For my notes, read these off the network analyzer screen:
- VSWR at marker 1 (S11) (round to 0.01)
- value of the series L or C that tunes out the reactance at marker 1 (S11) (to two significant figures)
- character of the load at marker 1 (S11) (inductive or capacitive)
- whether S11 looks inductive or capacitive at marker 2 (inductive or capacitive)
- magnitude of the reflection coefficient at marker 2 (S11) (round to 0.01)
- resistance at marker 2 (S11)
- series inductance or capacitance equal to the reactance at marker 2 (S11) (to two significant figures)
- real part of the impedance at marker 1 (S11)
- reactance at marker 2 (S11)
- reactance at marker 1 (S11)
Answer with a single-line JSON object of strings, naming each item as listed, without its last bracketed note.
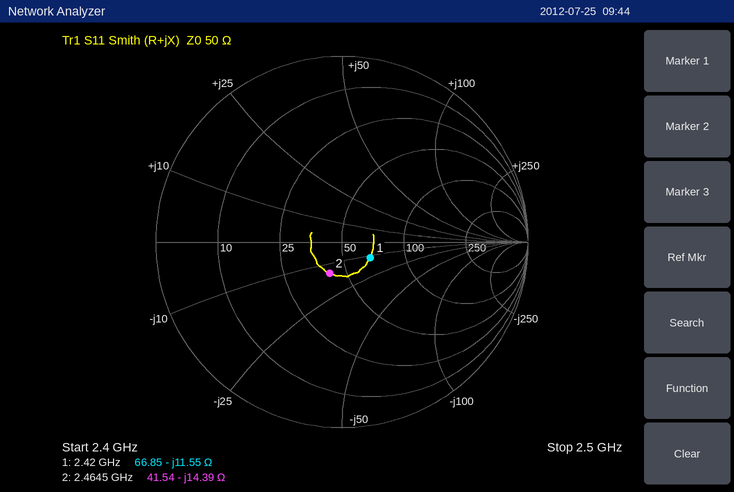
{"VSWR at marker 1 (S11)": "1.42", "value of the series L or C that tunes out the reactance at marker 1 (S11)": "760 pH", "character of the load at marker 1 (S11)": "capacitive", "whether S11 looks inductive or capacitive at marker 2": "capacitive", "magnitude of the reflection coefficient at marker 2 (S11)": "0.18", "resistance at marker 2": "41.54 Ω", "series inductance or capacitance equal to the reactance at marker 2 (S11)": "4.5 pF", "real part of the impedance at marker 1": "66.85 Ω", "reactance at marker 2": "-14.39 Ω", "reactance at marker 1": "-11.55 Ω"}
